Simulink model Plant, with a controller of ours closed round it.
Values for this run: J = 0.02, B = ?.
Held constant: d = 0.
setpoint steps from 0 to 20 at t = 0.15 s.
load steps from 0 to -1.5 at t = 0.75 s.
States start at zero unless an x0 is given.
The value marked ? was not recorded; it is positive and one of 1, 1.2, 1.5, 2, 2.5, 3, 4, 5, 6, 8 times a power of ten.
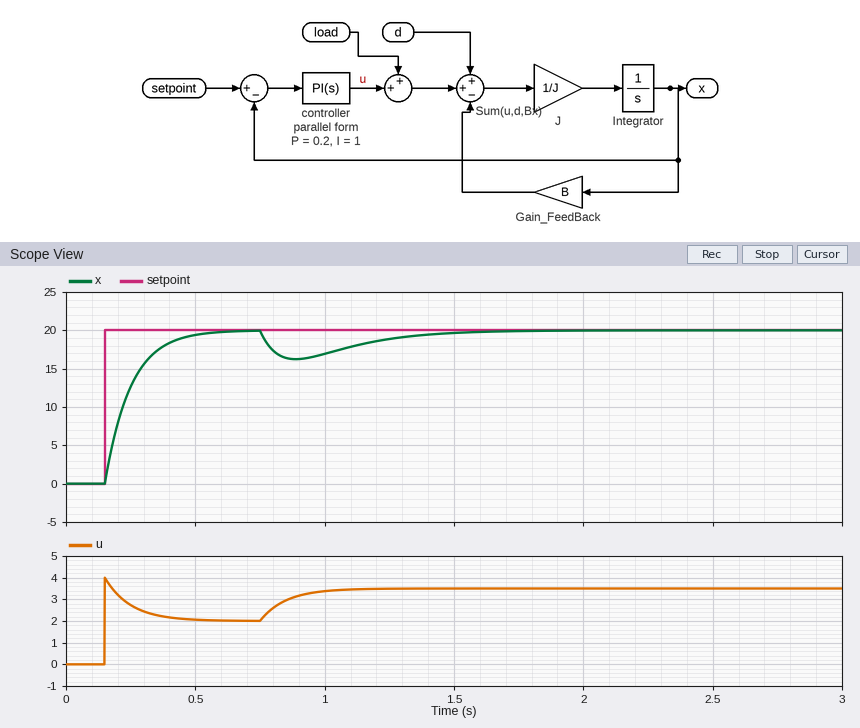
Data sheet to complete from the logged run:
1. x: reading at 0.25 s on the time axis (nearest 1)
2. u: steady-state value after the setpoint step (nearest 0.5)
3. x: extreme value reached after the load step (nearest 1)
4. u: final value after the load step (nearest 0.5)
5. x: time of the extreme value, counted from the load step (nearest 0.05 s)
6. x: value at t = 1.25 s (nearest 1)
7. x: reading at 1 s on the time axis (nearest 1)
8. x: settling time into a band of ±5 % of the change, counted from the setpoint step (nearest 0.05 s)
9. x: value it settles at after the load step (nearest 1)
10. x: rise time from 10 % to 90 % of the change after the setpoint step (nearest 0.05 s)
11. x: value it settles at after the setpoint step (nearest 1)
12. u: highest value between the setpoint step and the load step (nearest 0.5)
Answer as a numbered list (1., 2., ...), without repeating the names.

1. 13
2. 2.0
3. 16
4. 3.5
5. 0.15 s
6. 19
7. 17
8. 0.30 s
9. 20
10. 0.20 s
11. 20
12. 4.0
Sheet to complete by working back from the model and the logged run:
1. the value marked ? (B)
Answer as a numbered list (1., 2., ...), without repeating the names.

1. 0.1
